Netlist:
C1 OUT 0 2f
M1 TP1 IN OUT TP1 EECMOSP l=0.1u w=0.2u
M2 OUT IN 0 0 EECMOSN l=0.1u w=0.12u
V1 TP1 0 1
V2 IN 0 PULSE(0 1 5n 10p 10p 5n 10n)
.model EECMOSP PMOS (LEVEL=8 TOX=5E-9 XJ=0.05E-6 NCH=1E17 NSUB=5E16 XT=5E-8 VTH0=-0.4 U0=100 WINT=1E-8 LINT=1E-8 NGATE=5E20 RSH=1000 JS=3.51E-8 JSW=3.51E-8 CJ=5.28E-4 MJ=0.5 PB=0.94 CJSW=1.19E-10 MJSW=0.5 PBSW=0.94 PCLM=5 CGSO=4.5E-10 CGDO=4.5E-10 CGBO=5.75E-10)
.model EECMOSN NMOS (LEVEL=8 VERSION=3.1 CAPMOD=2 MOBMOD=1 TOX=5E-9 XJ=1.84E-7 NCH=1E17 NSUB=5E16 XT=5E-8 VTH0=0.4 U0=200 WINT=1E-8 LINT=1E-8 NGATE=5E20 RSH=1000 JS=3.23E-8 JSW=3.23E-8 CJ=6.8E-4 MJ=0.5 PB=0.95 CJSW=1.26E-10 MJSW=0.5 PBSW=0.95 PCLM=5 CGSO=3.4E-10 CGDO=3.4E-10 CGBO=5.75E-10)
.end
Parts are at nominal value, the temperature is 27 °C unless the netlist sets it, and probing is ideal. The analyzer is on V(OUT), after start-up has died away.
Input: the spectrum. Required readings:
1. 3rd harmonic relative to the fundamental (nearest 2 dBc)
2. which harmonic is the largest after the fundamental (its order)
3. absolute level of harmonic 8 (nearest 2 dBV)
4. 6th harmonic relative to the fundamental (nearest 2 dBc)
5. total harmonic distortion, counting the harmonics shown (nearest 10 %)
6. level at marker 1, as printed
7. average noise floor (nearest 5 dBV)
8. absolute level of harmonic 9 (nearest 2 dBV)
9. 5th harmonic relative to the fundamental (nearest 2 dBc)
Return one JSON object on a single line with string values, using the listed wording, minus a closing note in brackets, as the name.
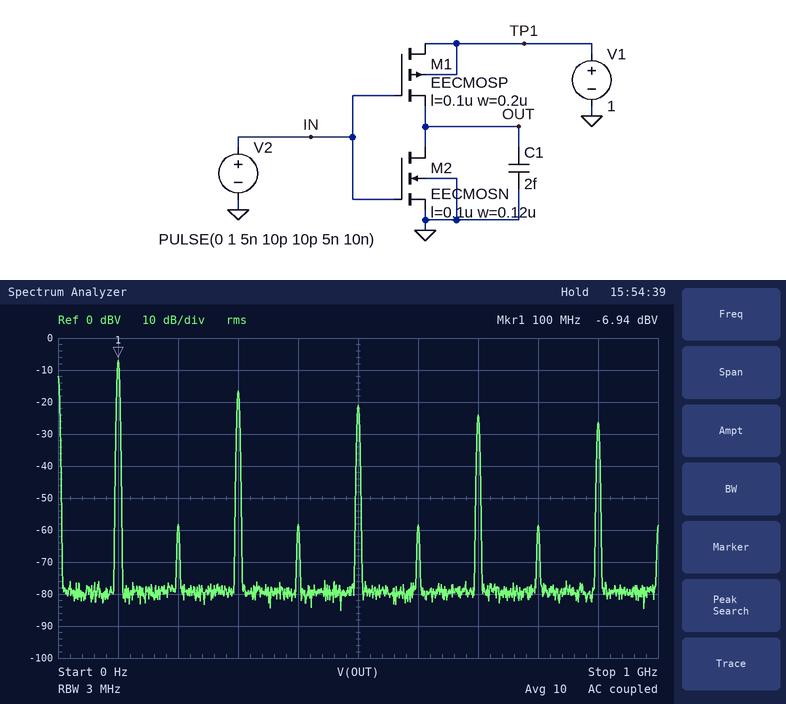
{"3rd harmonic relative to the fundamental": "-10 dBc", "which harmonic is the largest after the fundamental": "3", "absolute level of harmonic 8": "-58 dBV", "6th harmonic relative to the fundamental": "-52 dBc", "total harmonic distortion, counting the harmonics shown": "40 %", "level at marker 1, as printed": "-6.94 dBV", "average noise floor": "-80 dBV", "absolute level of harmonic 9": "-26 dBV", "5th harmonic relative to the fundamental": "-14 dBc"}
